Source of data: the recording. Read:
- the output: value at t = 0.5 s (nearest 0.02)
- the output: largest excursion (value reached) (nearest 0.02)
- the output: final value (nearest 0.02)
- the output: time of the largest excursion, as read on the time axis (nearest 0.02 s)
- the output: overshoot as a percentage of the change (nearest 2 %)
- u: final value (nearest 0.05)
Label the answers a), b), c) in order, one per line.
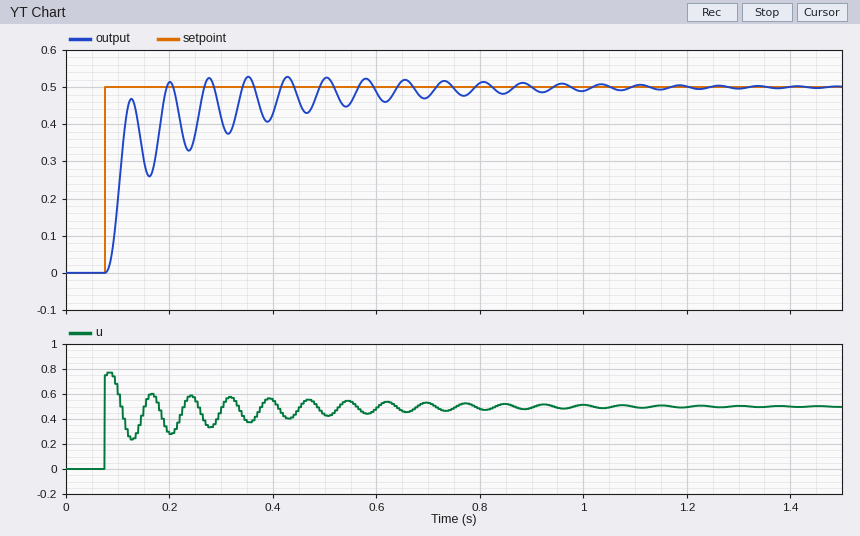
a) 0.52
b) 0.52
c) 0.50
d) 0.36 s
e) 6 %
f) 0.50
